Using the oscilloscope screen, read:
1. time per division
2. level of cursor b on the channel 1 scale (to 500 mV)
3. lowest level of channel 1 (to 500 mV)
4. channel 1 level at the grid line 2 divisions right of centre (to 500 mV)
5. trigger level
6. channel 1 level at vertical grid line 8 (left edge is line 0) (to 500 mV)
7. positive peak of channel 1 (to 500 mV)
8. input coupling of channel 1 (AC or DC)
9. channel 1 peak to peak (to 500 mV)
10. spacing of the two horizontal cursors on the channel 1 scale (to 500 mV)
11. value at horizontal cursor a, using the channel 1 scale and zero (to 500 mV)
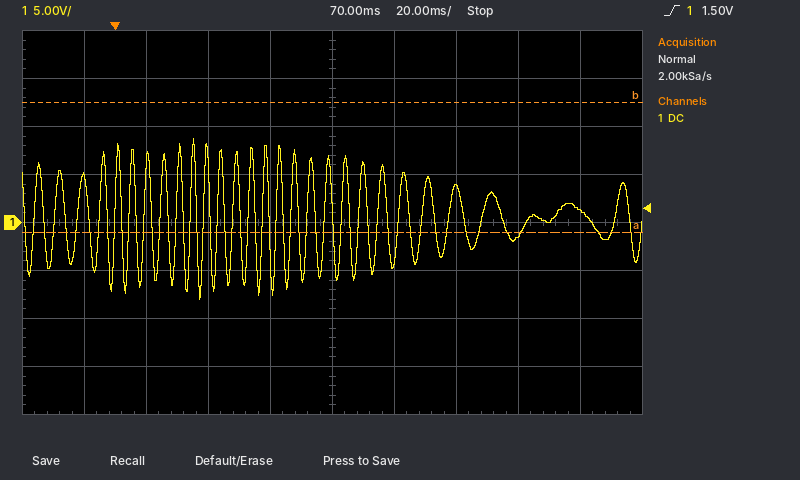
20 ms
12.5 V
-8.0 V
3.5 V
1.50 V
-1.5 V
9.0 V
DC
17.0 V
13.5 V
-1.0 V
